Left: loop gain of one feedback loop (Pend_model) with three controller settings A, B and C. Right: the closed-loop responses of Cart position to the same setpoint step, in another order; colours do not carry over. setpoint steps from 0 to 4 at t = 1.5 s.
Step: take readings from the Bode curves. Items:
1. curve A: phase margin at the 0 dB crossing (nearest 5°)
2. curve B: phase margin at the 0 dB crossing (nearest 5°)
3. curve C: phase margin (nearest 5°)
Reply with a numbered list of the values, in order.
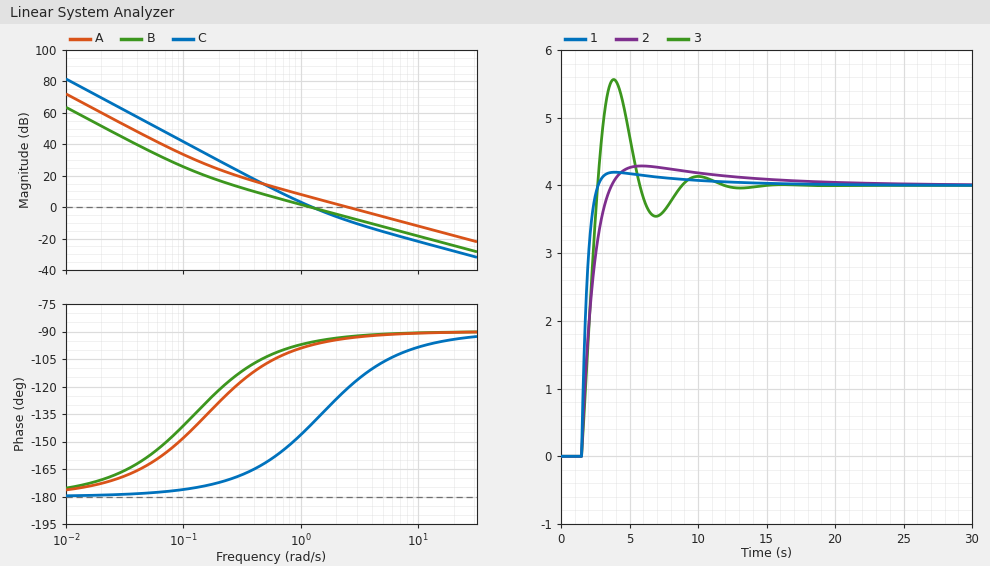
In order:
1. 85°
2. 85°
3. 40°
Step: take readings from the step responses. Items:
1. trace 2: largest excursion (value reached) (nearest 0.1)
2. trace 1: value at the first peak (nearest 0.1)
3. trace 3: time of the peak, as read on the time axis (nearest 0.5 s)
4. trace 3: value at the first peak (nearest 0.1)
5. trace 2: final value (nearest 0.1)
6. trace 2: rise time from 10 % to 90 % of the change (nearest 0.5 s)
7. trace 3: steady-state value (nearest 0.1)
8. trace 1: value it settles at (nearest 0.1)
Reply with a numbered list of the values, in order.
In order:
1. 4.3
2. 4.2
3. 4.0 s
4. 5.6
5. 4.0
6. 1.5 s
7. 4.0
8. 4.0
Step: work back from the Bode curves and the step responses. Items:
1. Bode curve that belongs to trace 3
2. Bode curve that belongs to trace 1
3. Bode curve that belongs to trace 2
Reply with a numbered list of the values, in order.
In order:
1. C
2. A
3. B
